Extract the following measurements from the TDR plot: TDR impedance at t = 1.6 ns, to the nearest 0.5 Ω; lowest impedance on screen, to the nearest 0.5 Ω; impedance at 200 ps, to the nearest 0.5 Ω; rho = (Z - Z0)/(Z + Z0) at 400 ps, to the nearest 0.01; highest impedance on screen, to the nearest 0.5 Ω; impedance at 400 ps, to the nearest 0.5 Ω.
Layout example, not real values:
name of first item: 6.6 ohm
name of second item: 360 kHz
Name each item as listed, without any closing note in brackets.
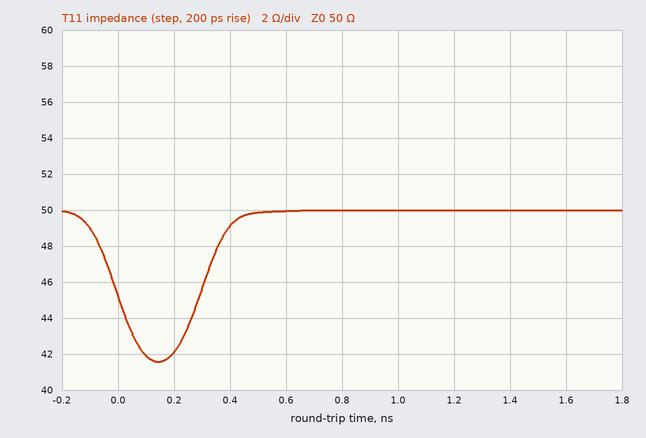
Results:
TDR impedance at t = 1.6 ns, to the nearest 0.5 Ω: 50.0 Ω
lowest impedance on screen, to the nearest 0.5 Ω: 41.5 Ω
impedance at 200 ps, to the nearest 0.5 Ω: 42.0 Ω
rho = (Z - Z0)/(Z + Z0) at 400 ps, to the nearest 0.01: -0.01
highest impedance on screen, to the nearest 0.5 Ω: 50.0 Ω
impedance at 400 ps, to the nearest 0.5 Ω: 49.0 Ω
